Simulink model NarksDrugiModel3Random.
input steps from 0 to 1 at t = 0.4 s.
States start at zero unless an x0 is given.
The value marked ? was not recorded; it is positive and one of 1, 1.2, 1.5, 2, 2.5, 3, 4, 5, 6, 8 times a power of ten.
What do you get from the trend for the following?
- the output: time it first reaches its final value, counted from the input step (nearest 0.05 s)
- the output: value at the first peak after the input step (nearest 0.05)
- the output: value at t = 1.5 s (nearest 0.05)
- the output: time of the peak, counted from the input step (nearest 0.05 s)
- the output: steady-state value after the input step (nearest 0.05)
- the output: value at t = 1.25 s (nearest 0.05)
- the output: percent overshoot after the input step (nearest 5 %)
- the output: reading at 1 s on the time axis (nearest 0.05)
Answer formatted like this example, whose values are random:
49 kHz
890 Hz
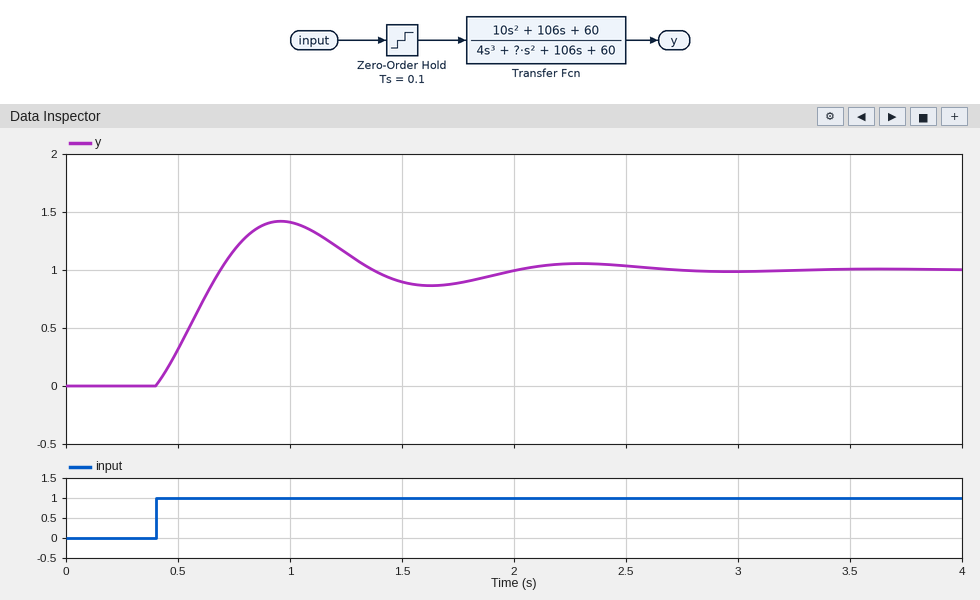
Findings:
0.30 s
1.40
0.90
0.55 s
1.00
1.15
40 %
1.40
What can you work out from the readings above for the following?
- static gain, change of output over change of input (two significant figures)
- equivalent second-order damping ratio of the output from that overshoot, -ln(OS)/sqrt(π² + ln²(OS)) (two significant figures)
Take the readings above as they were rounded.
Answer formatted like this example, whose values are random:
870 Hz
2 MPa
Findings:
1.0
0.28
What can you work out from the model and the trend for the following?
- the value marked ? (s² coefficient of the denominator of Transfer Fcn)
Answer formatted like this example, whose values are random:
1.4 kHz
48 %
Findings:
15
